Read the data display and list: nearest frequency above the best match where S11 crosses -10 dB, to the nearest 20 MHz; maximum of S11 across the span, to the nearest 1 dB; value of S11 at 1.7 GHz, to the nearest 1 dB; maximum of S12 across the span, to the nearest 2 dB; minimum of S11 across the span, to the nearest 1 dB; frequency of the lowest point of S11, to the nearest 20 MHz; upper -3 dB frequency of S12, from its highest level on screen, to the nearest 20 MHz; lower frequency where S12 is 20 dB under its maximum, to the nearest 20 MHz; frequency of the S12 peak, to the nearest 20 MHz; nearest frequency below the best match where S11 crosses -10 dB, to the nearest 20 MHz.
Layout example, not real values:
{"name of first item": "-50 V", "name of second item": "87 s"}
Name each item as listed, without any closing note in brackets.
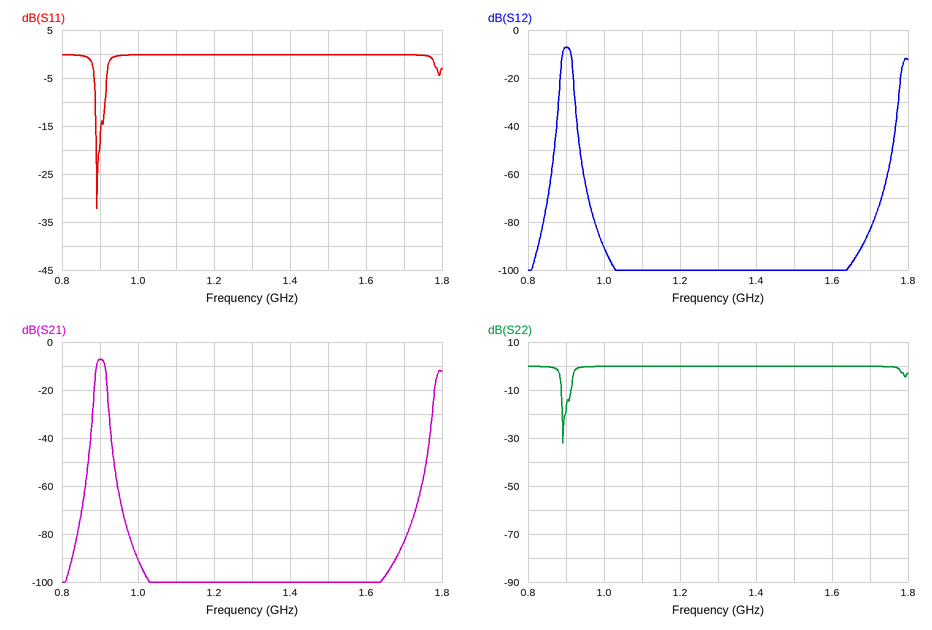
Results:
{"nearest frequency above the best match where S11 crosses -10 dB, to the nearest 20 MHz": "920 MHz", "maximum of S11 across the span, to the nearest 1 dB": "0 dB", "value of S11 at 1.7 GHz, to the nearest 1 dB": "0 dB", "maximum of S12 across the span, to the nearest 2 dB": "-8 dB", "minimum of S11 across the span, to the nearest 1 dB": "-32 dB", "frequency of the lowest point of S11, to the nearest 20 MHz": "900 MHz", "upper -3 dB frequency of S12, from its highest level on screen, to the nearest 20 MHz": "920 MHz", "lower frequency where S12 is 20 dB under its maximum, to the nearest 20 MHz": "880 MHz", "frequency of the S12 peak, to the nearest 20 MHz": "900 MHz", "nearest frequency below the best match where S11 crosses -10 dB, to the nearest 20 MHz": "880 MHz"}
